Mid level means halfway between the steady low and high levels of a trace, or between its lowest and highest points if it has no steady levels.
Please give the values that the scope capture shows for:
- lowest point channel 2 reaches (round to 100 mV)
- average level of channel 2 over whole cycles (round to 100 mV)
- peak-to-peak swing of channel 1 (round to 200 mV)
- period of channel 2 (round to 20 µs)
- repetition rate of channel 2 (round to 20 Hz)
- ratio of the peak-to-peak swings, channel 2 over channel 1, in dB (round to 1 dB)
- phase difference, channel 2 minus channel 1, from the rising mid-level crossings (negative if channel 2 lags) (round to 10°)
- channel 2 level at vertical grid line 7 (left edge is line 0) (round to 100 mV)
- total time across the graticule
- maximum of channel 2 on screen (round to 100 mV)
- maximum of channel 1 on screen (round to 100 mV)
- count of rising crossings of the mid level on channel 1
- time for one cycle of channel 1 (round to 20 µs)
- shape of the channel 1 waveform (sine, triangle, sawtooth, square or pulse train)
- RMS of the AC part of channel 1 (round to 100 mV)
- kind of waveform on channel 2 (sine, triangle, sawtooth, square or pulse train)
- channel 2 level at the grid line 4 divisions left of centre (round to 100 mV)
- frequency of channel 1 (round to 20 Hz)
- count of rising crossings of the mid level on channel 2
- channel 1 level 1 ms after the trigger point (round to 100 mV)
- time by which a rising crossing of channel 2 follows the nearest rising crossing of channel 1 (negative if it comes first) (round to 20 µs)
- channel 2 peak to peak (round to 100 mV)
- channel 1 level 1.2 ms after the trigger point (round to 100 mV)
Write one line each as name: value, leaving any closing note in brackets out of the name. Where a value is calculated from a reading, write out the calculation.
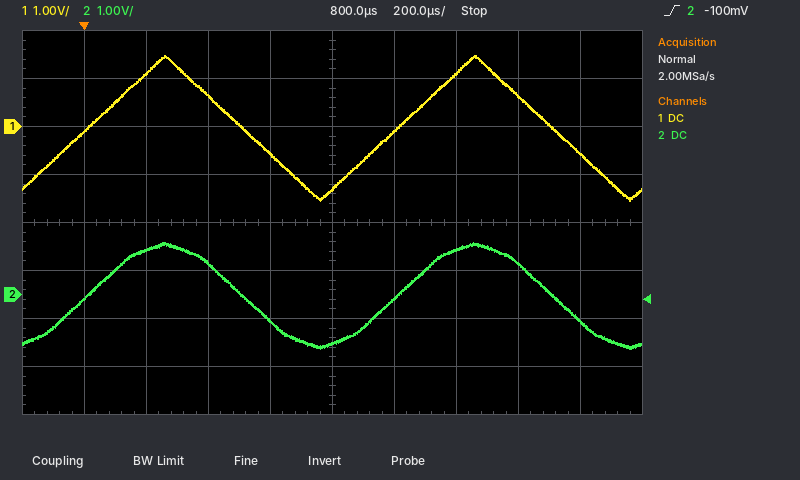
lowest point channel 2 reaches: -1.1 V
average level of channel 2 over whole cycles: (1.1 V + (-1.1 V)) / 2 ≈ 0.0 V
peak-to-peak swing of channel 1: 3.0 V
period of channel 2: 1.00 ms
repetition rate of channel 2: 1 / 1.00 ms ≈ 1.00 kHz
ratio of the peak-to-peak swings, channel 2 over channel 1, in dB: 20 log10(2.2 V / 3.0 V) ≈ -3 dB
phase difference, channel 2 minus channel 1, from the rising mid-level crossings (negative if channel 2 lags): −360° × (0 µs) / 1.00 ms ≈ 0°
channel 2 level at vertical grid line 7 (left edge is line 0): 900 mV
total time across the graticule: 2 ms
maximum of channel 2 on screen: 1.1 V
maximum of channel 1 on screen: 1.5 V
count of rising crossings of the mid level on channel 1: 2
time for one cycle of channel 1: 1.00 ms
shape of the channel 1 waveform: triangle
RMS of the AC part of channel 1: 3.0 V / (2√3) ≈ 866 mV, so 900 mV to the nearest 100 mV
kind of waveform on channel 2: sine
channel 2 level at the grid line 4 divisions left of centre: -100 mV
frequency of channel 1: 1 / 1.00 ms ≈ 1.00 kHz
count of rising crossings of the mid level on channel 2: 2
channel 1 level 1 ms after the trigger point: -100 mV
time by which a rising crossing of channel 2 follows the nearest rising crossing of channel 1 (negative if it comes first): 0 µs
channel 2 peak to peak: 1.1 V − (-1.1 V) = 2.2 V
channel 1 level 1.2 ms after the trigger point: 1.1 V
